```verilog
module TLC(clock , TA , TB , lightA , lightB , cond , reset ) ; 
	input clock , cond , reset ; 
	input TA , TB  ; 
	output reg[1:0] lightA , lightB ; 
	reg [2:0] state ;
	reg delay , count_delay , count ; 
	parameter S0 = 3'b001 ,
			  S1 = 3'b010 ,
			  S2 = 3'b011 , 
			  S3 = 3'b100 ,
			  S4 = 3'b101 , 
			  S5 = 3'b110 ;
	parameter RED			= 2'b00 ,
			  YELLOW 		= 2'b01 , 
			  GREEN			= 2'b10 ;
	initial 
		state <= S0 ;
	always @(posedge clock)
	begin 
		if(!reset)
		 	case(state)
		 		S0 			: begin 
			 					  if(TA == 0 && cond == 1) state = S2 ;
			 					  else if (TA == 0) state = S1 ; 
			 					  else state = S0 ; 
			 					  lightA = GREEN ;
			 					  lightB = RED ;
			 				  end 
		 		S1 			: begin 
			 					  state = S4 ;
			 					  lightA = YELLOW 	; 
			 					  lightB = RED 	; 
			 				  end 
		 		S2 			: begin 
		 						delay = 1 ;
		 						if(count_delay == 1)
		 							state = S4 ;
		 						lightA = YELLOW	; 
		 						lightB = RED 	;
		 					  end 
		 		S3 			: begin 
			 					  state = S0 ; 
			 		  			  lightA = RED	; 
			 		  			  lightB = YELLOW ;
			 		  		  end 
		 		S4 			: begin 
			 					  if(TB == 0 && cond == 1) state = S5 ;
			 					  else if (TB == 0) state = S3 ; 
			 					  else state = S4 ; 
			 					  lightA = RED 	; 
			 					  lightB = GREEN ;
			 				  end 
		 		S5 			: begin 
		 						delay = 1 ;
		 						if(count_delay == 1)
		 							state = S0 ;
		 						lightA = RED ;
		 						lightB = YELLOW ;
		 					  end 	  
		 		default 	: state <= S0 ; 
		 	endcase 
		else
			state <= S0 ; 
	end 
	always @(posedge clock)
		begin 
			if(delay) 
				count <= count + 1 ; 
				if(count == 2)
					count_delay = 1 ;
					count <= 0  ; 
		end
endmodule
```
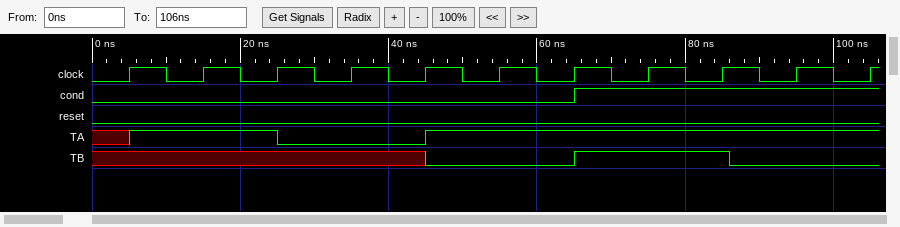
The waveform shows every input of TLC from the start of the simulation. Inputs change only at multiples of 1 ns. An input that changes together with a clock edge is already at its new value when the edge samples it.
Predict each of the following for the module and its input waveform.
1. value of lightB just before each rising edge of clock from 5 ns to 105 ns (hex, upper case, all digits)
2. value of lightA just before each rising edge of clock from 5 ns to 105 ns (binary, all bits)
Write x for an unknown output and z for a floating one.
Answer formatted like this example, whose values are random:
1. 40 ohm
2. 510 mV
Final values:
1. x, 0, 0, 0, 0, 2, 1, 0, 0, 0, 0
2. x, 10, 10, 10, 01, 00, 00, 10, 10, 10, 10
